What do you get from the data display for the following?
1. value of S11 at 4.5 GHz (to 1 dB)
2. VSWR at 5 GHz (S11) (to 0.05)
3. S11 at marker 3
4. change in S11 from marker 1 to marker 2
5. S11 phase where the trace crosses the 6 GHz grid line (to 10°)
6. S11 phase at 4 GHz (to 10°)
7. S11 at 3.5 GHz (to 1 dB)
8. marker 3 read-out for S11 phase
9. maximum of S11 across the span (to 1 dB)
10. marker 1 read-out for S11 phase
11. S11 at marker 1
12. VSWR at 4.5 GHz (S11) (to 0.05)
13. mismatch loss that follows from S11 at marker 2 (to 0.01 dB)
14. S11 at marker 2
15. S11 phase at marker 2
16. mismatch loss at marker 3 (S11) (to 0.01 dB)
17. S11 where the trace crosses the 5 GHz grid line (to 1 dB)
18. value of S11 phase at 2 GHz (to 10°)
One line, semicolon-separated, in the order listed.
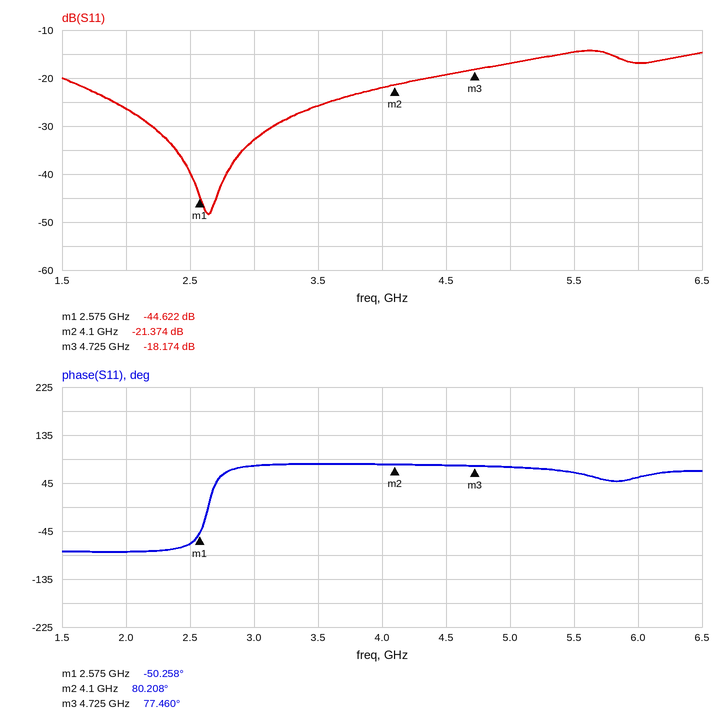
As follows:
-19 dB; 1.35; -18.174 dB; 23.248 dB; 60°; 80°; -26 dB; 77.460°; -14 dB; -50.258°; -44.622 dB; 1.25; 0.03 dB; -21.374 dB; 80.208°; 0.07 dB; -17 dB; -80°
